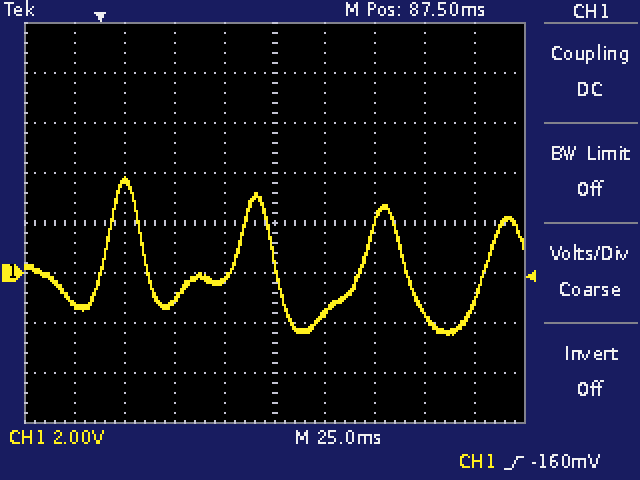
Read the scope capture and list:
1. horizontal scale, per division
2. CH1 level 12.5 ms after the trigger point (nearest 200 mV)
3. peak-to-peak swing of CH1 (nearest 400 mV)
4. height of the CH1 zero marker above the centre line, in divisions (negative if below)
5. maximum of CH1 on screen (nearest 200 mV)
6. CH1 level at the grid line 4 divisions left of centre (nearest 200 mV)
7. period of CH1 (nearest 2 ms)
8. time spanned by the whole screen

25 ms
3.6 V
6.4 V
-1.0 div
3.8 V
-1.2 V
64 ms
250 ms
